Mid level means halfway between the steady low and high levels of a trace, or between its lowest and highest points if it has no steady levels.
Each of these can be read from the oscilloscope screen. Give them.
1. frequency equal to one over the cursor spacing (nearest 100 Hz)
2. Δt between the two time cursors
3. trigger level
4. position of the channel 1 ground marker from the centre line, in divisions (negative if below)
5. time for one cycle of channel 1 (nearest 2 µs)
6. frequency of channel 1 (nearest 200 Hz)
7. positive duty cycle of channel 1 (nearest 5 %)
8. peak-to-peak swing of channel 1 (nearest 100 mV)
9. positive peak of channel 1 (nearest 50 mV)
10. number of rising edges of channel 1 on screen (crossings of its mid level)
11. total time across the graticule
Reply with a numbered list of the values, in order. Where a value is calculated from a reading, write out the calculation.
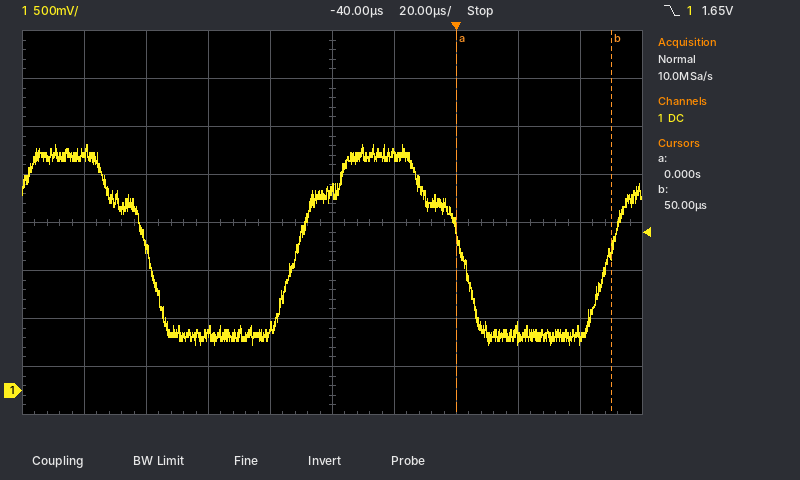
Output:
1. 1 / 50 µs ≈ 20.0 kHz
2. 50 µs − (0 s) = 50 µs
3. 1.65 V
4. -3.5 div
5. 102 µs
6. 1 / 102 µs ≈ 9.8 kHz
7. 50 %
8. 2.10 V
9. 2.55 V
10. 2
11. 200 µs
